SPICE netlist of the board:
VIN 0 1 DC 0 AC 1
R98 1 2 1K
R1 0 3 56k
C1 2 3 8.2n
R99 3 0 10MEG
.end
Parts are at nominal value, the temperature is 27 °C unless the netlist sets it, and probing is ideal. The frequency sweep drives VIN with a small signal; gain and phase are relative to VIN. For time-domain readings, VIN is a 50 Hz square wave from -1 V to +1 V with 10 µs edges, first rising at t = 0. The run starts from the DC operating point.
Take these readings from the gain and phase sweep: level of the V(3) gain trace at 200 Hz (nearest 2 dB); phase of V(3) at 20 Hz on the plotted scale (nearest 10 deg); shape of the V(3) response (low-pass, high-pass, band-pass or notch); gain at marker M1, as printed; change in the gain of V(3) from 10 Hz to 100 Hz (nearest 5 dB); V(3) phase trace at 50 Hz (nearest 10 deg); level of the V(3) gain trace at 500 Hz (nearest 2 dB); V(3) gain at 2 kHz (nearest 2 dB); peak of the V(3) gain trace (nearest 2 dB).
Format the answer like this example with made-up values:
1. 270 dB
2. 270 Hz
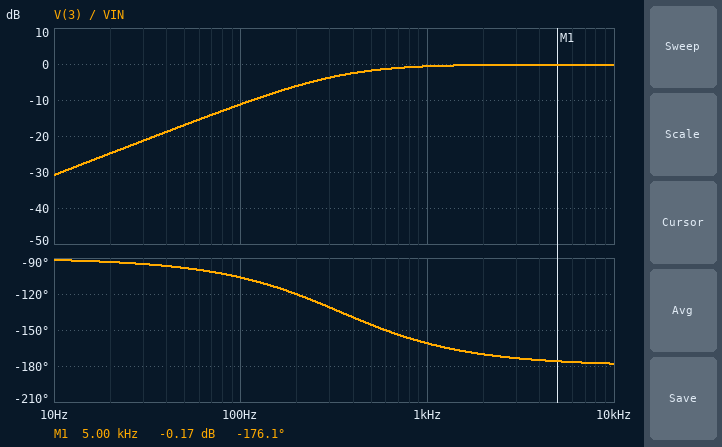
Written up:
1. -6 dB
2. -90 deg
3. high-pass
4. -0.17 dB
5. 20 dB
6. -100 deg
7. -2 dB
8. 0 dB
9. 0 dB
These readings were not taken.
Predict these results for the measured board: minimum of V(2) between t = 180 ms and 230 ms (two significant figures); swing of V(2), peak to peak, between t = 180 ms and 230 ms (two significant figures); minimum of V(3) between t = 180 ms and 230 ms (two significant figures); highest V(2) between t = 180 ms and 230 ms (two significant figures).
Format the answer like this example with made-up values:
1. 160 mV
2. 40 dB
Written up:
1. -1.0 V
2. 2.0 V
3. -1.9 V
4. 1.0 V
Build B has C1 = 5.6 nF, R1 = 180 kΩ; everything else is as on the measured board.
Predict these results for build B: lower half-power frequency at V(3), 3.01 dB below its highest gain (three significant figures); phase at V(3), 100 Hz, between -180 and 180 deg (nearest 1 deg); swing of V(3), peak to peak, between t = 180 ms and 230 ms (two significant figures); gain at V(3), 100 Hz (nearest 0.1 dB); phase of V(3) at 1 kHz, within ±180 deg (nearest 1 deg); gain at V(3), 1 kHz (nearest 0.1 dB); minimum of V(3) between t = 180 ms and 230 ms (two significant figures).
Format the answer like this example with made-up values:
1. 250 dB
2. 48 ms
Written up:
1. 160 Hz
2. -122 deg
3. 4.0 V
4. -5.6 dB
5. -171 deg
6. -0.2 dB
7. -2.0 V
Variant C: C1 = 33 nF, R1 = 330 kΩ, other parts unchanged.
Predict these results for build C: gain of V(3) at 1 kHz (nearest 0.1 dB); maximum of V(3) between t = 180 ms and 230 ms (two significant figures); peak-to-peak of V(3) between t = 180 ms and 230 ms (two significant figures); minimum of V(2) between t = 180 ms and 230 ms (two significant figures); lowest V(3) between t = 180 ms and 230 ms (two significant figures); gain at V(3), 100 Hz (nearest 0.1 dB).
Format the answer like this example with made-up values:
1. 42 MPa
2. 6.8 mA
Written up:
1. 0 dB
2. 1.4 V
3. 2.9 V
4. -1.0 V
5. -1.4 V
6. -0.1 dB
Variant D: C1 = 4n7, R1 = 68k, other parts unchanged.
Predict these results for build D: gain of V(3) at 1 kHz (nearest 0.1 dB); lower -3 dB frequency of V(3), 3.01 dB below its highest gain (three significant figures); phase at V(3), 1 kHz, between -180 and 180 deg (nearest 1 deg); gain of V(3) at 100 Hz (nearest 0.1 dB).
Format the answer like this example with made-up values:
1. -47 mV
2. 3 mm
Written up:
1. -1.1 dB
2. 494 Hz
3. -154 deg
4. -14.2 dB
